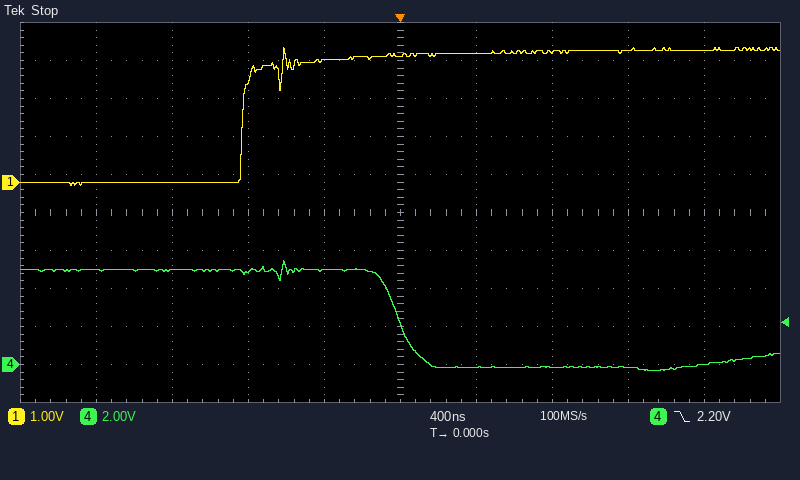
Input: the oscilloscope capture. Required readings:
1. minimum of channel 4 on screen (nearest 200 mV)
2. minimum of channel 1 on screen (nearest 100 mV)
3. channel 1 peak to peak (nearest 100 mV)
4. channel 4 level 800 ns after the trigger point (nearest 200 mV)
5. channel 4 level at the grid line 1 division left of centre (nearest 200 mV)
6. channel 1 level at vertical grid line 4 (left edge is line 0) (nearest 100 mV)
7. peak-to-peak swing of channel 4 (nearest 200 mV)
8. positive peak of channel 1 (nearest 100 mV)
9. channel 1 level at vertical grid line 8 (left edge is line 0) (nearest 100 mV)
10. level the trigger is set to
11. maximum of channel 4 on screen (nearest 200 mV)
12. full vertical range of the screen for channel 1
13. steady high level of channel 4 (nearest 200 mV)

-400 mV
-100 mV
3.6 V
-200 mV
5.0 V
3.2 V
5.8 V
3.5 V
3.5 V
2.20 V
5.4 V
10 V
5.0 V
